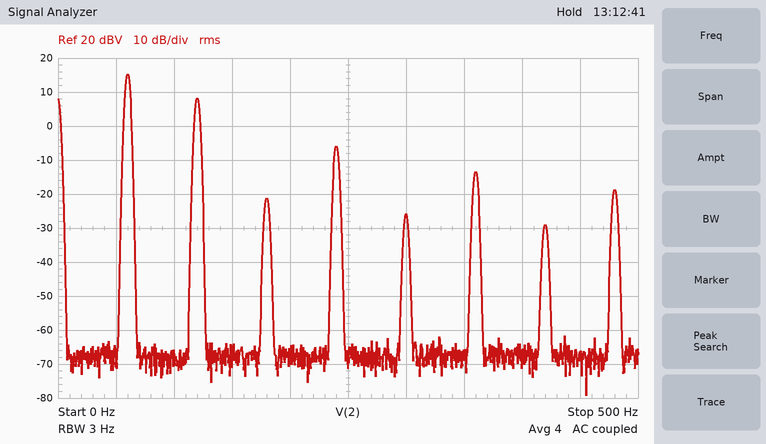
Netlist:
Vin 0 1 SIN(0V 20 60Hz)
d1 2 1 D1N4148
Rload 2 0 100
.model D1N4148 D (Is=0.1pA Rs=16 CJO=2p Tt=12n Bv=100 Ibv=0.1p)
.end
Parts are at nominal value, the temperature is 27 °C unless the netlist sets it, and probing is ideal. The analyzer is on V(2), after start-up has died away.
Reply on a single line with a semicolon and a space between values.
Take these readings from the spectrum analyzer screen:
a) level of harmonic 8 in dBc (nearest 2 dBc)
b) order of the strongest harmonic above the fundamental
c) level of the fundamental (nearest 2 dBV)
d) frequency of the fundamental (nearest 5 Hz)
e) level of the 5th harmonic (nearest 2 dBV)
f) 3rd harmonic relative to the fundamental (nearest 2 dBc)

-34 dBc; 2; 16 dBV; 60 Hz; -26 dBV; -36 dBc
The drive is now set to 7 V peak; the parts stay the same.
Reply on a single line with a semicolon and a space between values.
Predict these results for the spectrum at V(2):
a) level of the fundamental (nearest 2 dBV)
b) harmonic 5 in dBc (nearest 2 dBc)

6 dBV; -32 dBc
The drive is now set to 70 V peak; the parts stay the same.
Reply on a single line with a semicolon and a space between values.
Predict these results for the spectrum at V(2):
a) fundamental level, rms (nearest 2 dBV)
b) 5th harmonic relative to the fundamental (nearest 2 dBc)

26 dBV; -52 dBc
